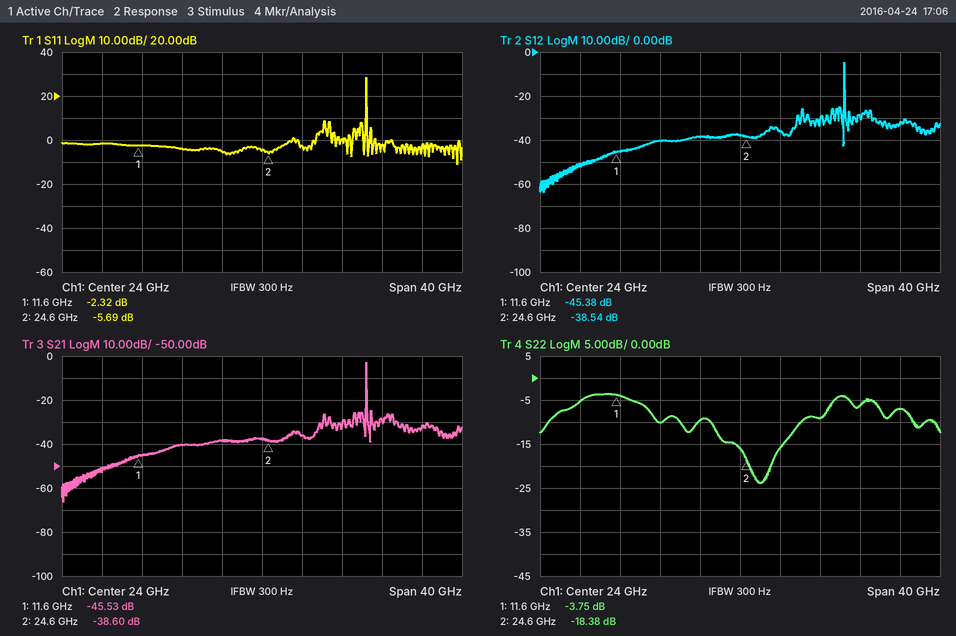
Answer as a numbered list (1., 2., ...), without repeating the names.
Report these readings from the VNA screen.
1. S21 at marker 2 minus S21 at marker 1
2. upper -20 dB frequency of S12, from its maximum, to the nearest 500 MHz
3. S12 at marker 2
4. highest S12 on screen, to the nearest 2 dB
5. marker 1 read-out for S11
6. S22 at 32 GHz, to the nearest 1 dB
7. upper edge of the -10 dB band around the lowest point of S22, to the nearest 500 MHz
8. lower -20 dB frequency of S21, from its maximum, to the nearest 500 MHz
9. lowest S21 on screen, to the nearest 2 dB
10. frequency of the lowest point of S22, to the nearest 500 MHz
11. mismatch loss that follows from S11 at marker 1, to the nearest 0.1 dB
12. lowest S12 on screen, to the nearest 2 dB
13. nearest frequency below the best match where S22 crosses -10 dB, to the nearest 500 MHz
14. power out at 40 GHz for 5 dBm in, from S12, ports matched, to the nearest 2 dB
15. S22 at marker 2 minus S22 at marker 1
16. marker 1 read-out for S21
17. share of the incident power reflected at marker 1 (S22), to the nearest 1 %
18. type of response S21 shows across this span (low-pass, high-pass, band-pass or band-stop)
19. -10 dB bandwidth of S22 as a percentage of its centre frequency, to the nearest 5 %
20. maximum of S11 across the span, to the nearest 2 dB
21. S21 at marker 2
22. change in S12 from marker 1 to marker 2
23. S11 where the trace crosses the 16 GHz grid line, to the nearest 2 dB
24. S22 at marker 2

1. 6.93 dB
2. 34.5 GHz
3. -38.54 dB
4. -4 dB
5. -2.32 dB
6. -9 dB
7. 30.0 GHz
8. 34.5 GHz
9. -66 dB
10. 26.0 GHz
11. 3.8 dB
12. -64 dB
13. 21.0 GHz
14. -28 dBm
15. -14.63 dB
16. -45.53 dB
17. 42 %
18. band-pass
19. 35 %
20. 28 dB
21. -38.60 dB
22. 6.84 dB
23. -4 dB
24. -18.38 dB
